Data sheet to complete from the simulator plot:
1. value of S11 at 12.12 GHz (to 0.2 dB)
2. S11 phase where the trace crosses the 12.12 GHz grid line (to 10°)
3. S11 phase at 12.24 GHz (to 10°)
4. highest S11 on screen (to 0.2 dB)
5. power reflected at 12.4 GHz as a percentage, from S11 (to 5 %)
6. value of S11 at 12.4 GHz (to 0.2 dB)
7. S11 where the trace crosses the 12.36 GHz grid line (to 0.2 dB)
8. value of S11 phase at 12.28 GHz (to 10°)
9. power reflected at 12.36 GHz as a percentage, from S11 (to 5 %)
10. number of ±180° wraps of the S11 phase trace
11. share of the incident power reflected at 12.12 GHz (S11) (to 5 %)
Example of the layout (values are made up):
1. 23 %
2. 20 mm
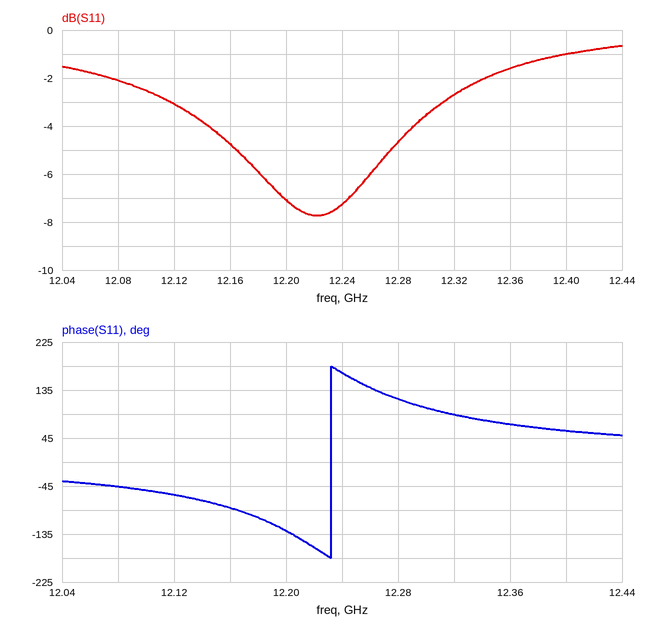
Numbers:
1. -3.0 dB
2. -60°
3. 170°
4. -0.6 dB
5. 80 %
6. -1.0 dB
7. -1.6 dB
8. 120°
9. 70 %
10. 1
11. 50 %
